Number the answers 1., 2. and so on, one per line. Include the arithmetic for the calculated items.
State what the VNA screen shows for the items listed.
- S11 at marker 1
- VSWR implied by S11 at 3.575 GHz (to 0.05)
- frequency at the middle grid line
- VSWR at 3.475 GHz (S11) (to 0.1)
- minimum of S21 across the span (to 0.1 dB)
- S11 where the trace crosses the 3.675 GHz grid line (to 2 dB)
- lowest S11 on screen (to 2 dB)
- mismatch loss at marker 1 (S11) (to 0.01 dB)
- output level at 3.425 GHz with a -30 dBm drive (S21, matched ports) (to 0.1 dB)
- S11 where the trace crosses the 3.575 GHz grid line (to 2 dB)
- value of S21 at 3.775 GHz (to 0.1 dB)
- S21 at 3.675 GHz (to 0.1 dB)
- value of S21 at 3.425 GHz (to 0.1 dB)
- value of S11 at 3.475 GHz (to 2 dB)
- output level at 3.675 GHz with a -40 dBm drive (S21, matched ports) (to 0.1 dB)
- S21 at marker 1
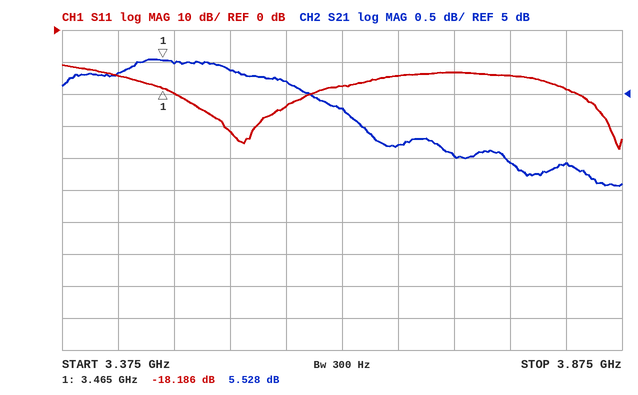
1. -18.186 dB
2. |Γ| = 10^(-24/20) = 0.0631; VSWR = (1 + 0.0631)/(1 − 0.0631) ≈ 1.13, so 1.15 to the nearest 0.05
3. 3.625 GHz
4. |Γ| = 10^(-20/20) = 0.1000; VSWR = (1 + 0.1000)/(1 − 0.1000) ≈ 1.2
5. 3.6 dB
6. -14 dB
7. -38 dB
8. −10 log10(1 − 10^(-18.186/10)) ≈ 0.07 dB
9. -30 dBm + (5.3 dB) = -24.7 dBm
10. -24 dB
11. 3.9 dB
12. 4.2 dB
13. 5.3 dB
14. -20 dB
15. -40 dBm + (4.2 dB) = -35.8 dBm
16. 5.528 dB
